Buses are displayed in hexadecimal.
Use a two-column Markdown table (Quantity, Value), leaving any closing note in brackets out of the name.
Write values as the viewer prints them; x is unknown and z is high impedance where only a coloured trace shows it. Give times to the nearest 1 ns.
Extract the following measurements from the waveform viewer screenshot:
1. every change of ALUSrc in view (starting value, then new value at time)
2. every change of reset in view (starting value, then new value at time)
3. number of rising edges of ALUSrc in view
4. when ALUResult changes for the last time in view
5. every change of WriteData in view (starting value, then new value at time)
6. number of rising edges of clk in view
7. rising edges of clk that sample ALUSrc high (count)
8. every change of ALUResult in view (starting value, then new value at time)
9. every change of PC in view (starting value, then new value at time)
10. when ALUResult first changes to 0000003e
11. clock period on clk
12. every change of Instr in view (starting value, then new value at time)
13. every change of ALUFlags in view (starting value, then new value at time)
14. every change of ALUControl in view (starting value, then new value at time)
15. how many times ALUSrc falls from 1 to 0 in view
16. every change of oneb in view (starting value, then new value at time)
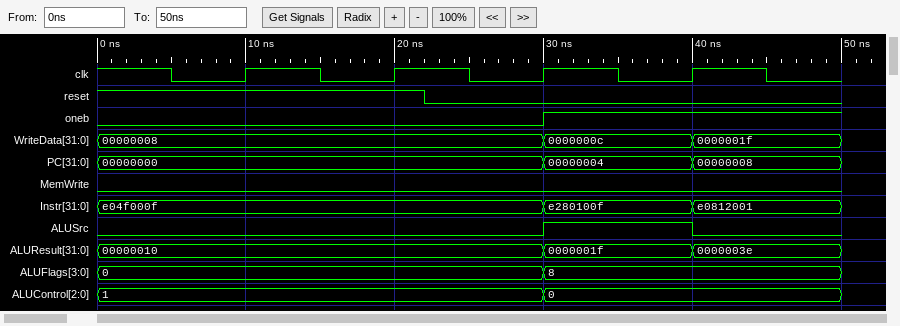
| Quantity | Value |
|---|---|
| every change of ALUSrc in view | 0, 1 at 30 ns, 0 at 40 ns |
| every change of reset in view | 1, 0 at 22 ns |
| number of rising edges of ALUSrc in view | 1 |
| when ALUResult changes for the last time in view | 40 ns |
| every change of WriteData in view | 00000008, 0000000c at 30 ns, 0000001f at 40 ns |
| number of rising edges of clk in view | 4 |
| rising edges of clk that sample ALUSrc high | 1 |
| every change of ALUResult in view | 00000010, 0000001f at 30 ns, 0000003e at 40 ns |
| every change of PC in view | 00000000, 00000004 at 30 ns, 00000008 at 40 ns |
| when ALUResult first changes to 0000003e | 40 ns |
| clock period on clk | 10 ns |
| every change of Instr in view | e04f000f, e280100f at 30 ns, e0812001 at 40 ns |
| every change of ALUFlags in view | 0, 8 at 30 ns |
| every change of ALUControl in view | 1, 0 at 30 ns |
| how many times ALUSrc falls from 1 to 0 in view | 1 |
| every change of oneb in view | 0, 1 at 30 ns |
